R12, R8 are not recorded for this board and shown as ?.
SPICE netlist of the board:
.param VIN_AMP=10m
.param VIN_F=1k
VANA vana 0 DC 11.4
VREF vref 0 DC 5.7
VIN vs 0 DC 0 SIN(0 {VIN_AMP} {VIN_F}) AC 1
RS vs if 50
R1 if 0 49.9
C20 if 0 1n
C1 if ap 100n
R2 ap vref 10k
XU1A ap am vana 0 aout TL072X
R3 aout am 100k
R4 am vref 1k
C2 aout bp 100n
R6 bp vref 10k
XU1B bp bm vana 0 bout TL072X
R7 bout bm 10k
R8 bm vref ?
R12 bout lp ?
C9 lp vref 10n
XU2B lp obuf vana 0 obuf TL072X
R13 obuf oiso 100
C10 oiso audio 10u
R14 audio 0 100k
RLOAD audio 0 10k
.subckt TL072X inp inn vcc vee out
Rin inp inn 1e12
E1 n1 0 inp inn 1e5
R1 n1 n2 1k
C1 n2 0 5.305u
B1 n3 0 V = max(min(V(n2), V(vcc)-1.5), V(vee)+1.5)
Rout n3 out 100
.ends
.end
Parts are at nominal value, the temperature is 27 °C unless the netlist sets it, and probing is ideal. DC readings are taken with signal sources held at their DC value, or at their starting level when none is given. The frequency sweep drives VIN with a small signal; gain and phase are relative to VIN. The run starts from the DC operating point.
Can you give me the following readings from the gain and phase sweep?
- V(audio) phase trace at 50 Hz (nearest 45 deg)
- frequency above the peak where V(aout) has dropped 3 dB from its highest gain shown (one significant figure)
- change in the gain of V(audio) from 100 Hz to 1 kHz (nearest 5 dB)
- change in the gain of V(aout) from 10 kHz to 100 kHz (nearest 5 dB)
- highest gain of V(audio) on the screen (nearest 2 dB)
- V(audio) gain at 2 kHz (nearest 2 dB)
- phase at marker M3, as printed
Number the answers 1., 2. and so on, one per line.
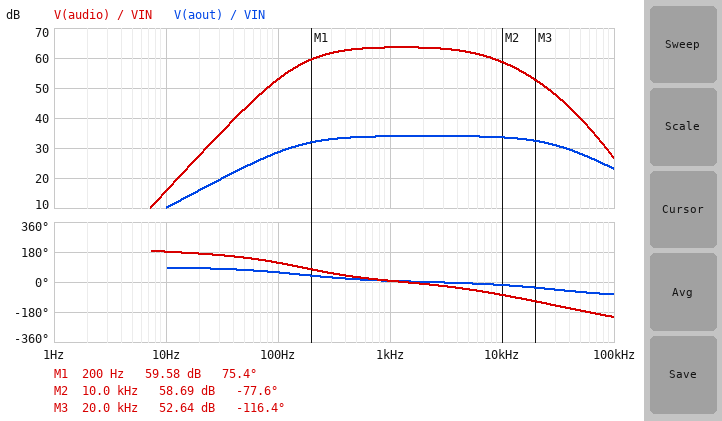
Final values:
1. 135 deg
2. 30 kHz
3. 10 dB
4. -10 dB
5. 64 dB
6. 64 dB
7. -116.4 deg
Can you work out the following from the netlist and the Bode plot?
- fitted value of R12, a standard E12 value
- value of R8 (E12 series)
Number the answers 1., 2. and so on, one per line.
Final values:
1. 2.2 kΩ
2. 330 Ω
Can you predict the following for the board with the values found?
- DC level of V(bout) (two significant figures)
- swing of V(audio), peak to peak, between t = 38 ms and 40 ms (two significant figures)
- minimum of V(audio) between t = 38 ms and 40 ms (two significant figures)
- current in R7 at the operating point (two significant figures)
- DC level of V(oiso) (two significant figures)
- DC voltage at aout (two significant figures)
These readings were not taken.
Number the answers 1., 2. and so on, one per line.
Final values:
1. 5.7 V
2. 8.2 V
3. -4.1 V
4. 170 nA
5. 5.7 V
6. 5.7 V
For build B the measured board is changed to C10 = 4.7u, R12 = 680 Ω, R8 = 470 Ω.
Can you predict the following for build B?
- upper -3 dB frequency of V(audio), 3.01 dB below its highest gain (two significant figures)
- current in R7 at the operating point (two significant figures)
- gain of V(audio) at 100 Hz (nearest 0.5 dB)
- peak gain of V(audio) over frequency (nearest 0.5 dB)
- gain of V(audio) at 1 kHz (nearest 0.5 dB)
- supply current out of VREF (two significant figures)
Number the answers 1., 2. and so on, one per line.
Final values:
1. 17 kHz
2. 120 nA
3. 50.0 dB
4. 61.0 dB
5. 60.5 dB
6. 180 nA
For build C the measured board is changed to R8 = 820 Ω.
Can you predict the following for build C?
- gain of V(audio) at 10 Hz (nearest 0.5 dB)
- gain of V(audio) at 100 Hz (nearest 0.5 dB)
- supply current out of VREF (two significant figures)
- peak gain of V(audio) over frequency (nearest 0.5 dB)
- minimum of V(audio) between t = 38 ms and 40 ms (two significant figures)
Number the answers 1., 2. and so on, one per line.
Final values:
1. 8.0 dB
2. 45.5 dB
3. 130 nA
4. 56.0 dB
5. -4.1 V
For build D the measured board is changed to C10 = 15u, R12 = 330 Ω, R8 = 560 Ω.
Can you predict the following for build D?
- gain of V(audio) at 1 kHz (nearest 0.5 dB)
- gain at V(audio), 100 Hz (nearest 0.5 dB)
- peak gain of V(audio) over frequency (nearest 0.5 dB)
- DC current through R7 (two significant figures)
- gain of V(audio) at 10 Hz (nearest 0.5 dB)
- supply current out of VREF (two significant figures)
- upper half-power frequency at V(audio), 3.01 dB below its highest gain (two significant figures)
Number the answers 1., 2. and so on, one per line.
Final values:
1. 59.0 dB
2. 48.5 dB
3. 59.5 dB
4. 100 nA
5. 11.5 dB
6. 160 nA
7. 24 kHz
